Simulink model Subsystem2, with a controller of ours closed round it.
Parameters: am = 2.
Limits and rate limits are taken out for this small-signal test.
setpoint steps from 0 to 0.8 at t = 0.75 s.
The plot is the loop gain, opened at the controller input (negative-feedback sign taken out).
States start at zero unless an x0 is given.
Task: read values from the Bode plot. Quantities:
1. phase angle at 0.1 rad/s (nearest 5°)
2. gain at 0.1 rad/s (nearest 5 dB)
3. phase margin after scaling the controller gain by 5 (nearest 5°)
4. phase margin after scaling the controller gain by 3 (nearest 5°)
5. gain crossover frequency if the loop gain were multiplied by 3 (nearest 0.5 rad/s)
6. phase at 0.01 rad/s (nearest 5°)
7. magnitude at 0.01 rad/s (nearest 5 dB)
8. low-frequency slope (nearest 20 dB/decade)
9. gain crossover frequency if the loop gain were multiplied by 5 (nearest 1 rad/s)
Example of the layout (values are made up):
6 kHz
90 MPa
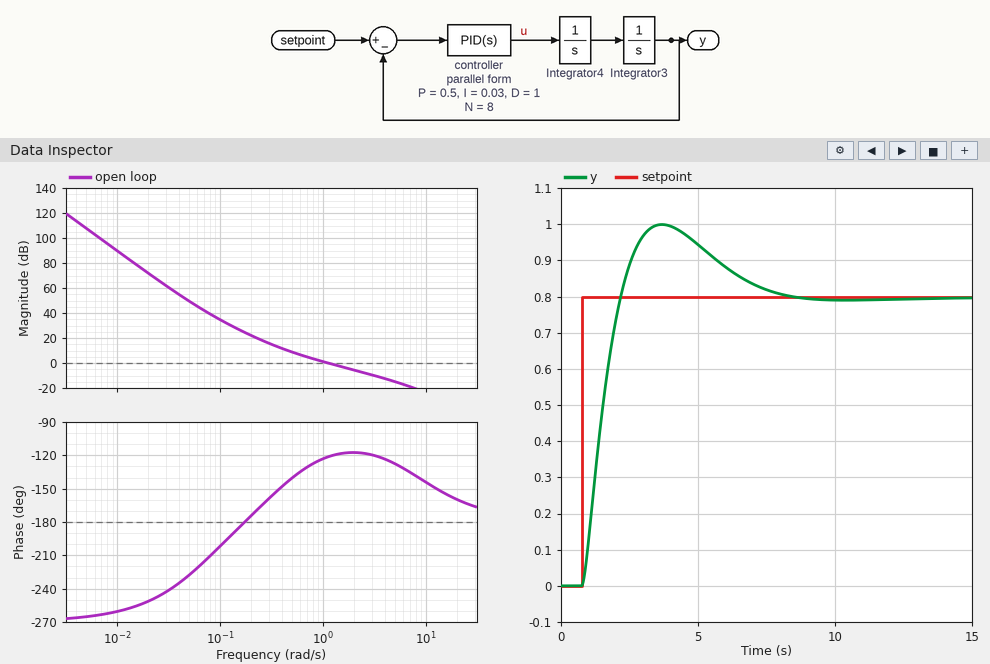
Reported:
-200°
35 dB
55°
60°
3.0 rad/s
-260°
90 dB
-60 dB/decade
5 rad/s
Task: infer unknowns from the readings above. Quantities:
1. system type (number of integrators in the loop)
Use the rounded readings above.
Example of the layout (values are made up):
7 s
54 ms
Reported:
3
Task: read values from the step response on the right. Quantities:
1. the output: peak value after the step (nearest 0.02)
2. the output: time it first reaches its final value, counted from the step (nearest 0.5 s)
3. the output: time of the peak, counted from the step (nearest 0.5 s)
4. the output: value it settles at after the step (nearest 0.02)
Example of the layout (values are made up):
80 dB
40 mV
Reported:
1.00
1.5 s
3.0 s
0.80
